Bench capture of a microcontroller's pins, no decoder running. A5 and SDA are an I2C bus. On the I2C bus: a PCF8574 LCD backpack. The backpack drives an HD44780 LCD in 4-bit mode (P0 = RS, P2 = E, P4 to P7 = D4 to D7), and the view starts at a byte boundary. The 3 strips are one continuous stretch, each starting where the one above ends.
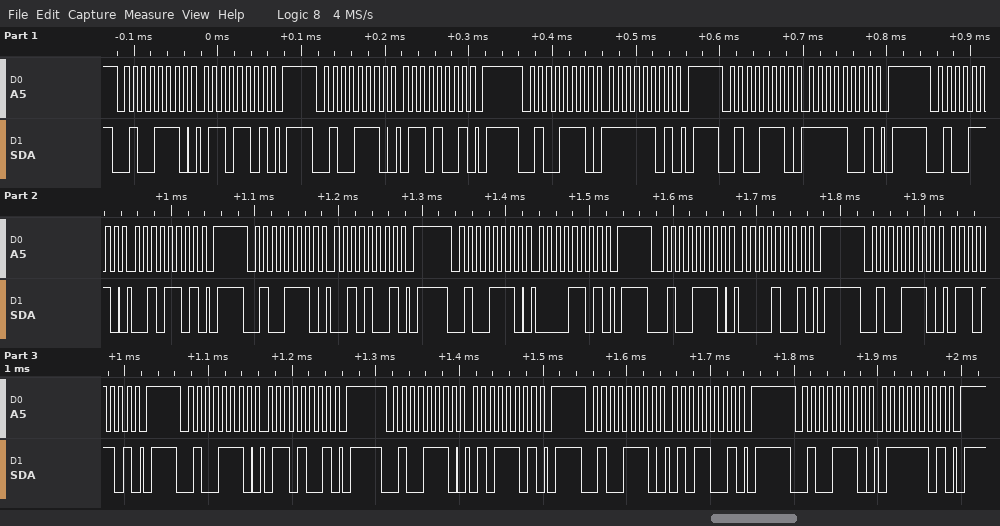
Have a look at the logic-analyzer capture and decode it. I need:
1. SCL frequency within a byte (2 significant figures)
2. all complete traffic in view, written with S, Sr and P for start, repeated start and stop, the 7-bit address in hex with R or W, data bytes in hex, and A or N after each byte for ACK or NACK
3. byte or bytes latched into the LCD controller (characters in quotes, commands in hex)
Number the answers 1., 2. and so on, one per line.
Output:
1. 100 kHz
2. S 27W A 6D A P S 27W A 69 A P S 27W A FD A P S 27W A F9 A P S 27W A 2D A P S 27W A 29 A P S 27W A 0D A P S 27W A 09 A P S 27W A 6D A P S 27W A 69 A P S 27W A 5D A P S 27W A 59 A P S 27W A 7D A P
3. 'o' ' ' 'e'
